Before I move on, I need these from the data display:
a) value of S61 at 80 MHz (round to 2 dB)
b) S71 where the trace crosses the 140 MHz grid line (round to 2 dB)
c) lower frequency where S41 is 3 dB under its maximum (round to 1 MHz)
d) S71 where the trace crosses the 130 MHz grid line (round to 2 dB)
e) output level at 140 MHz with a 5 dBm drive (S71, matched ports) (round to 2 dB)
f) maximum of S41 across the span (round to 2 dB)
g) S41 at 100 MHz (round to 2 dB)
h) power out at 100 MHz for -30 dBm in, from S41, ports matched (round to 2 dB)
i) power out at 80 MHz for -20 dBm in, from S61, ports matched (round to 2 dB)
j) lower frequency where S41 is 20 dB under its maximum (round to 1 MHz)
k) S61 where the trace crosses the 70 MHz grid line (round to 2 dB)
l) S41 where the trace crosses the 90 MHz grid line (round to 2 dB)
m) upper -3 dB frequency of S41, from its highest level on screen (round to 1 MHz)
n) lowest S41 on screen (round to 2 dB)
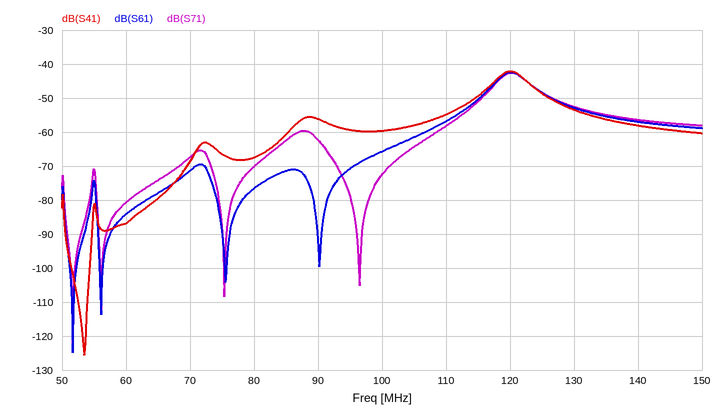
-76 dB
-56 dB
118 MHz
-52 dB
-52 dBm
-42 dB
-60 dB
-90 dBm
-96 dBm
84 MHz
-72 dB
-56 dB
123 MHz
-126 dB
